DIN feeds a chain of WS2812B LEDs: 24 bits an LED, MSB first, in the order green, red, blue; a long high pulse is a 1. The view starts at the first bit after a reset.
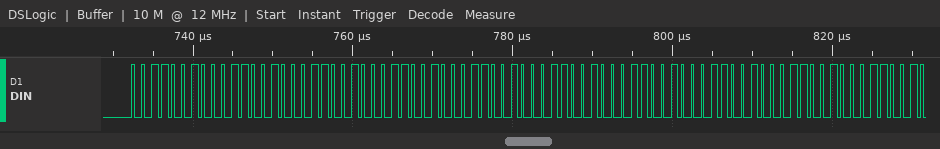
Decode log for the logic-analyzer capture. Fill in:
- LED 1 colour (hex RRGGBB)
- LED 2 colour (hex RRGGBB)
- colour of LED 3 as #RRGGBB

#323232
#323232
#323232
